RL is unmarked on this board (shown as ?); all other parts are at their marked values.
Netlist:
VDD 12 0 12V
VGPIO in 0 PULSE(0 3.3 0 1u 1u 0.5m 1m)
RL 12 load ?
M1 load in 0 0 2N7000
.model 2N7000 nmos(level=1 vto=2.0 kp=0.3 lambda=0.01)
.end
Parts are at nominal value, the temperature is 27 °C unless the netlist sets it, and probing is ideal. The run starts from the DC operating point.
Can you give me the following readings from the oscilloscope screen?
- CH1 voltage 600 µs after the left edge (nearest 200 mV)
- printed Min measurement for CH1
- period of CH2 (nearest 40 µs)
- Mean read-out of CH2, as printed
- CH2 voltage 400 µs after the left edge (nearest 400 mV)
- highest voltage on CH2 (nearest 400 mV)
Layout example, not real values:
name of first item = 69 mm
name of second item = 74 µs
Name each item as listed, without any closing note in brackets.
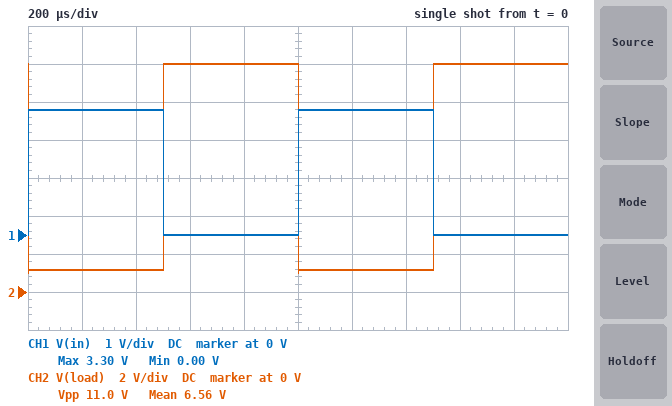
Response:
CH1 voltage 600 µs after the left edge = 0 V
printed Min measurement for CH1 = 0.00 V
period of CH2 = 1.00 ms
Mean read-out of CH2, as printed = 6.56 V
CH2 voltage 400 µs after the left edge = 1.2 V
highest voltage on CH2 = 12.0 V
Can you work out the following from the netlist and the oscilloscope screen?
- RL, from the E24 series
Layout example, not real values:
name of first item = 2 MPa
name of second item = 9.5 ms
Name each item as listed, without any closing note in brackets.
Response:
RL, from the E24 series = 43 Ω
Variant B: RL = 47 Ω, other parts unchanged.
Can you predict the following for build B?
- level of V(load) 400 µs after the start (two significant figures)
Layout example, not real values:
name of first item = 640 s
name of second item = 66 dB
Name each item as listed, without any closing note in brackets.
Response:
level of V(load) 400 µs after the start = 930 mV
